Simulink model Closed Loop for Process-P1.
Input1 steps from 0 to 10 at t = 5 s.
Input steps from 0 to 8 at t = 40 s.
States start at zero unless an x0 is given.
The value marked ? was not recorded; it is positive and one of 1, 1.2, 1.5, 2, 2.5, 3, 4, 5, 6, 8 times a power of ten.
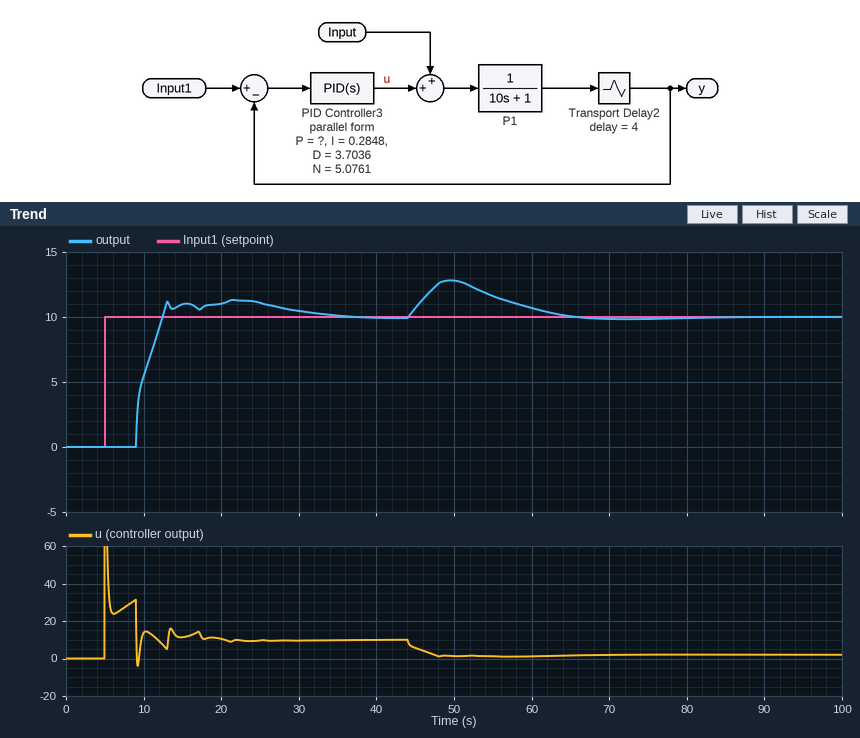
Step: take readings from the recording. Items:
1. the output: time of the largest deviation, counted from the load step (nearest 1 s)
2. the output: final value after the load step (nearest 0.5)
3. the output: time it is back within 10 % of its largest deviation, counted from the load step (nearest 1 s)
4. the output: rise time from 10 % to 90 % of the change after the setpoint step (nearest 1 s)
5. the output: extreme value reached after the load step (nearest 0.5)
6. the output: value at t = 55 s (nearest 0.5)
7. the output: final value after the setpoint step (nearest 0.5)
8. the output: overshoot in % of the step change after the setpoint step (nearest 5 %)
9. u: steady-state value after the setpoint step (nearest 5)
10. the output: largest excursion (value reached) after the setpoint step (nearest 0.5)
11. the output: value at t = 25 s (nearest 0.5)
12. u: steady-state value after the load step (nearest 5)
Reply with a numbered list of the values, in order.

1. 10 s
2. 10.0
3. 23 s
4. 3 s
5. 13.0
6. 11.5
7. 10.0
8. 15 %
9. 10
10. 11.5
11. 11.0
12. 0
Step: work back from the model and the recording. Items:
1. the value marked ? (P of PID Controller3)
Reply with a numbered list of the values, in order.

1. 2
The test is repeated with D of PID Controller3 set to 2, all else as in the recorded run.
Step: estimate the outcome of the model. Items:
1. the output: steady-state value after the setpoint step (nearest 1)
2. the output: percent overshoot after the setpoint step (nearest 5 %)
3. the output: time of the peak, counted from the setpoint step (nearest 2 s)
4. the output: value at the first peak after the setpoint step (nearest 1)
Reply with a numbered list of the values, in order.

1. 10
2. 25 %
3. 12 s
4. 13
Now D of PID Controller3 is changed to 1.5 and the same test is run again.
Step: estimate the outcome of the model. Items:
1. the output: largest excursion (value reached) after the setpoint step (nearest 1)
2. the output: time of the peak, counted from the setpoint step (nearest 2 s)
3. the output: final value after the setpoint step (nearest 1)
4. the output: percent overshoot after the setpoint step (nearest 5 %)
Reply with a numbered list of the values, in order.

1. 13
2. 12 s
3. 10
4. 30 %
